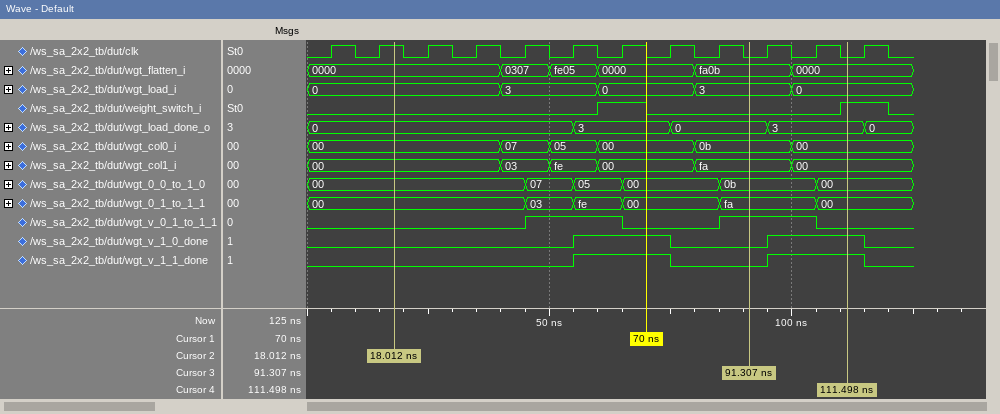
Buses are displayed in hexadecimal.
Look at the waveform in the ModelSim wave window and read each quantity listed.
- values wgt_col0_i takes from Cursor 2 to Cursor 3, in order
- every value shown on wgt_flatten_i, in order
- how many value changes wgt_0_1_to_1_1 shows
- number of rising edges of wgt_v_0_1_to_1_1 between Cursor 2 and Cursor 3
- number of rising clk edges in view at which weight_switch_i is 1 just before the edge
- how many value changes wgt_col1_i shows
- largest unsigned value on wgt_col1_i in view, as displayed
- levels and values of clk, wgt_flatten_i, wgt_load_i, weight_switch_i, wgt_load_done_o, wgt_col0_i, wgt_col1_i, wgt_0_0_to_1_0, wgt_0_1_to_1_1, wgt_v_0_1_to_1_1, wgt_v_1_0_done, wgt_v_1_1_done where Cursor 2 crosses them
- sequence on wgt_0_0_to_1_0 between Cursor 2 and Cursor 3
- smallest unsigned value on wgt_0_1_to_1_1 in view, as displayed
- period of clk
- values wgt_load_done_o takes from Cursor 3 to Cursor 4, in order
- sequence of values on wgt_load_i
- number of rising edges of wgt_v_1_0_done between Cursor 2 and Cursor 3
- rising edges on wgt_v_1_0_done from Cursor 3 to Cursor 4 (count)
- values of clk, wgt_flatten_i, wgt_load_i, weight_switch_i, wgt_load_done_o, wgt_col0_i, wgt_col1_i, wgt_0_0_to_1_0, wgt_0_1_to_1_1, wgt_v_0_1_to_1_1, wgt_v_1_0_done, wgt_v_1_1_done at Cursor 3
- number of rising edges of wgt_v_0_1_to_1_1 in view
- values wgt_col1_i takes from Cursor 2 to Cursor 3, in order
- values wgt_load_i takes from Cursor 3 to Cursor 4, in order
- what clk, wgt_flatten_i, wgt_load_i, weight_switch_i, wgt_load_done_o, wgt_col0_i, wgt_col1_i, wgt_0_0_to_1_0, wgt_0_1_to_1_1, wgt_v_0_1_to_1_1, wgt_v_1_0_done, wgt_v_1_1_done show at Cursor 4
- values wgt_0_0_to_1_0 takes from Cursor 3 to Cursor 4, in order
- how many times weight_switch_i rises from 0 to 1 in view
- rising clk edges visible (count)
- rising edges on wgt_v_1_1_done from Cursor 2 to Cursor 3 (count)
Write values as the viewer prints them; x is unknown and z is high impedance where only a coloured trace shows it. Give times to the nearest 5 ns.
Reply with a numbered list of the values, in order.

1. 00, 07, 05, 00, 0b
2. 0000, 0307, fe05, 0000, fa0b, 0000
3. 5
4. 2
5. 2
6. 5
7. fe
8. clk=1, wgt_flatten_i=0000, wgt_load_i=0, weight_switch_i=0, wgt_load_done_o=0, wgt_col0_i=00, wgt_col1_i=00, wgt_0_0_to_1_0=00, wgt_0_1_to_1_1=00, wgt_v_0_1_to_1_1=0, wgt_v_1_0_done=0, wgt_v_1_1_done=0
9. 00, 07, 05, 00, 0b
10. 00
11. 10 ns
12. 0, 3
13. 0, 3, 0, 3, 0
14. 1
15. 1
16. clk=0, wgt_flatten_i=fa0b, wgt_load_i=3, weight_switch_i=0, wgt_load_done_o=0, wgt_col0_i=0b, wgt_col1_i=fa, wgt_0_0_to_1_0=0b, wgt_0_1_to_1_1=fa, wgt_v_0_1_to_1_1=1, wgt_v_1_0_done=0, wgt_v_1_1_done=0
17. 2
18. 00, 03, fe, 00, fa
19. 3, 0
20. clk=0, wgt_flatten_i=0000, wgt_load_i=0, weight_switch_i=1, wgt_load_done_o=3, wgt_col0_i=00, wgt_col1_i=00, wgt_0_0_to_1_0=00, wgt_0_1_to_1_1=00, wgt_v_0_1_to_1_1=0, wgt_v_1_0_done=1, wgt_v_1_1_done=1
21. 0b, 00
22. 2
23. 12
24. 1
